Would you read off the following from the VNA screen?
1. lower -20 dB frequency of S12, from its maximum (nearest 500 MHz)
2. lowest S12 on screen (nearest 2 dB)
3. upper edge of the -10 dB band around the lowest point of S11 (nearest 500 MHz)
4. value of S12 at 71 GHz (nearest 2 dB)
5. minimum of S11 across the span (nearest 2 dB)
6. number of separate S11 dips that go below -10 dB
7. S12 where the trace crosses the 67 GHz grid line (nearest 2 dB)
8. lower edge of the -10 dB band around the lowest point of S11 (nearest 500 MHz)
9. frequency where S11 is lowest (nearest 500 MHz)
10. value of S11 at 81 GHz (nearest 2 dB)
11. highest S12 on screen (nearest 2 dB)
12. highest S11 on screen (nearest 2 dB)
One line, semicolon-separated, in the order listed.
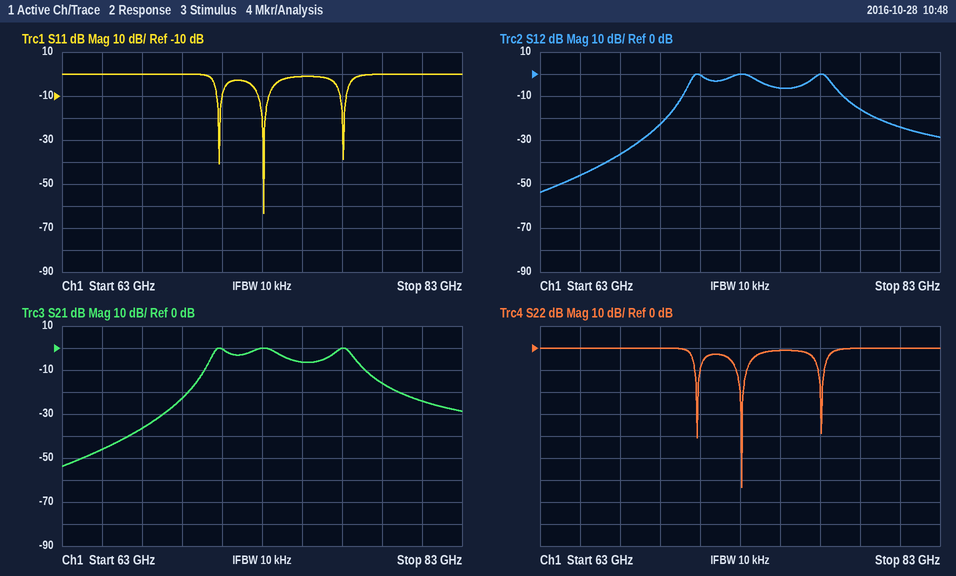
69.5 GHz; -54 dB; 73.5 GHz; 0 dB; -64 dB; 3; -36 dB; 73.0 GHz; 73.0 GHz; 0 dB; 0 dB; 0 dB
